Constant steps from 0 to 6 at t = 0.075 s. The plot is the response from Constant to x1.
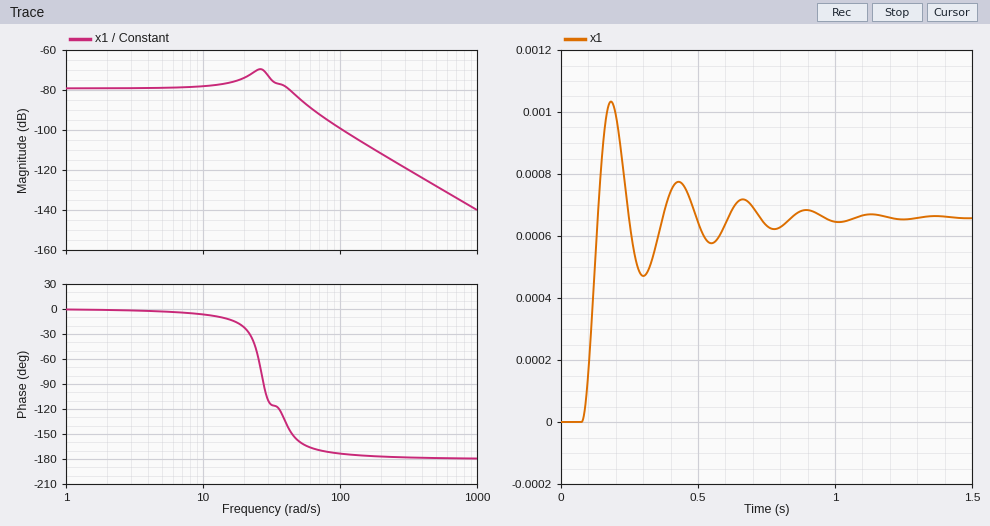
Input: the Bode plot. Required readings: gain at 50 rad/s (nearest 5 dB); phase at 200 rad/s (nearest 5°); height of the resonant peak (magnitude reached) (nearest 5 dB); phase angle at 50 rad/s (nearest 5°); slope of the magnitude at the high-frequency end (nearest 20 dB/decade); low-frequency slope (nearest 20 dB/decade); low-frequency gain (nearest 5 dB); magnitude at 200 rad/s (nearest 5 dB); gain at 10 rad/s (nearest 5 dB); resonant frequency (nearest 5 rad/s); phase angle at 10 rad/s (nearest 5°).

-85 dB
-175°
-70 dB
-160°
-40 dB/decade
0 dB/decade
-80 dB
-110 dB
-80 dB
25 rad/s
-5°
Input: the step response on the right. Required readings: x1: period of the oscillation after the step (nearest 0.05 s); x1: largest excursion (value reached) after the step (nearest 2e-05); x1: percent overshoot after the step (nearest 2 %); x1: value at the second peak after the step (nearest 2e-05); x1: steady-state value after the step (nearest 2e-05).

0.25 s
0.00104
56 %
0.00078
0.00066
